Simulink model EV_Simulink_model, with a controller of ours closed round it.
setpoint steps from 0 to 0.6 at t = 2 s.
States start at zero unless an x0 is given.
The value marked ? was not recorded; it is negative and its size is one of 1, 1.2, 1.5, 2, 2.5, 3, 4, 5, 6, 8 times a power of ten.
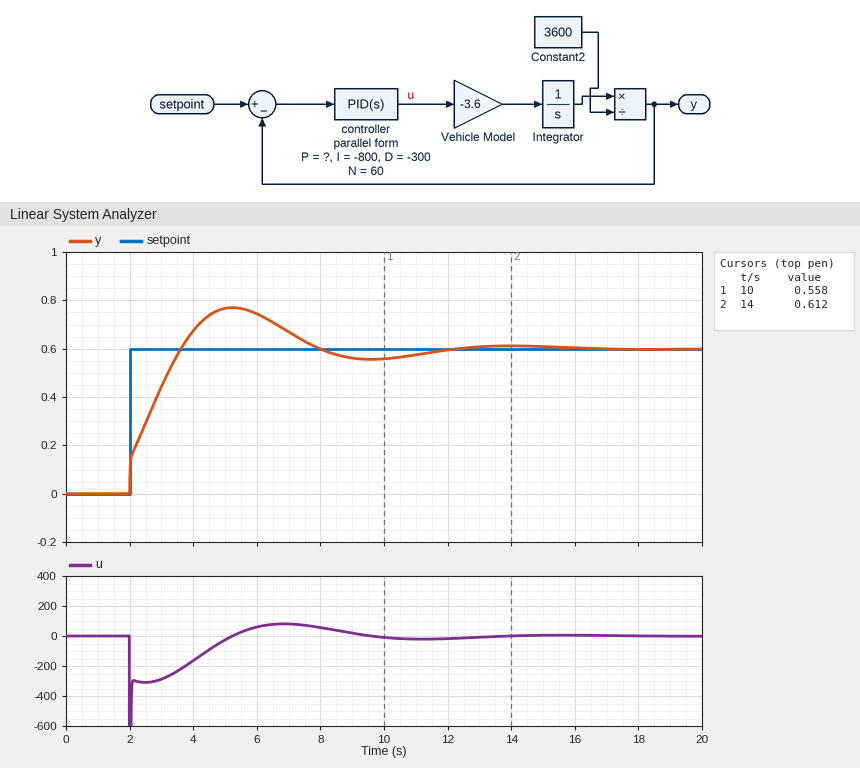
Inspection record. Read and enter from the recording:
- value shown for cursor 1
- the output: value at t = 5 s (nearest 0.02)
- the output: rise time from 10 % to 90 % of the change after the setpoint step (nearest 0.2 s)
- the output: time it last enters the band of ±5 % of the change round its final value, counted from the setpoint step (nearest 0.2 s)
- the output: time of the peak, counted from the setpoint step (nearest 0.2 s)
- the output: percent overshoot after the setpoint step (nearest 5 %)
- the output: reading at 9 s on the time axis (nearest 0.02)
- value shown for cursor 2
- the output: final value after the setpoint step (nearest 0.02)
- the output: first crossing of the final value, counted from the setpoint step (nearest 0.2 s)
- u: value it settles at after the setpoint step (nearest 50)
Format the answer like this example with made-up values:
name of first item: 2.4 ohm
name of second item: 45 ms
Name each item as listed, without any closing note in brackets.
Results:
value shown for cursor 1: 0.558
the output: value at t = 5 s: 0.76
the output: rise time from 10 % to 90 % of the change after the setpoint step: 1.4 s
the output: time it last enters the band of ±5 % of the change round its final value, counted from the setpoint step: 8.8 s
the output: time of the peak, counted from the setpoint step: 3.2 s
the output: percent overshoot after the setpoint step: 30 %
the output: reading at 9 s on the time axis: 0.56
value shown for cursor 2: 0.612
the output: final value after the setpoint step: 0.60
the output: first crossing of the final value, counted from the setpoint step: 1.6 s
u: value it settles at after the setpoint step: 0
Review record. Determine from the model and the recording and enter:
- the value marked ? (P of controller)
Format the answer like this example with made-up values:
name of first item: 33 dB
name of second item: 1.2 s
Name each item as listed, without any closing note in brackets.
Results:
the value marked ?: -800
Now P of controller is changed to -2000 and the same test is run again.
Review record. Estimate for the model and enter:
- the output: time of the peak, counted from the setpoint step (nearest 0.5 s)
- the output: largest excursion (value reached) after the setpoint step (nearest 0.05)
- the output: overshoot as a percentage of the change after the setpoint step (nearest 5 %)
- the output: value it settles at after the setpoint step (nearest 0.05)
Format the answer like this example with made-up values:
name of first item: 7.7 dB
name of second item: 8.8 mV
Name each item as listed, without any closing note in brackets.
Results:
the output: time of the peak, counted from the setpoint step: 2.5 s
the output: largest excursion (value reached) after the setpoint step: 0.65
the output: overshoot as a percentage of the change after the setpoint step: 10 %
the output: value it settles at after the setpoint step: 0.60
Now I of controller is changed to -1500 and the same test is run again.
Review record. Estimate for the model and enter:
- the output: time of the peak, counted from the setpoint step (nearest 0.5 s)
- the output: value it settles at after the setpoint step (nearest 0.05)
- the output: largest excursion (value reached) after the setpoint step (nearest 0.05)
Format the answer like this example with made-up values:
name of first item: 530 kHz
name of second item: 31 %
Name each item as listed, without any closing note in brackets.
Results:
the output: time of the peak, counted from the setpoint step: 2.5 s
the output: value it settles at after the setpoint step: 0.60
the output: largest excursion (value reached) after the setpoint step: 0.80
